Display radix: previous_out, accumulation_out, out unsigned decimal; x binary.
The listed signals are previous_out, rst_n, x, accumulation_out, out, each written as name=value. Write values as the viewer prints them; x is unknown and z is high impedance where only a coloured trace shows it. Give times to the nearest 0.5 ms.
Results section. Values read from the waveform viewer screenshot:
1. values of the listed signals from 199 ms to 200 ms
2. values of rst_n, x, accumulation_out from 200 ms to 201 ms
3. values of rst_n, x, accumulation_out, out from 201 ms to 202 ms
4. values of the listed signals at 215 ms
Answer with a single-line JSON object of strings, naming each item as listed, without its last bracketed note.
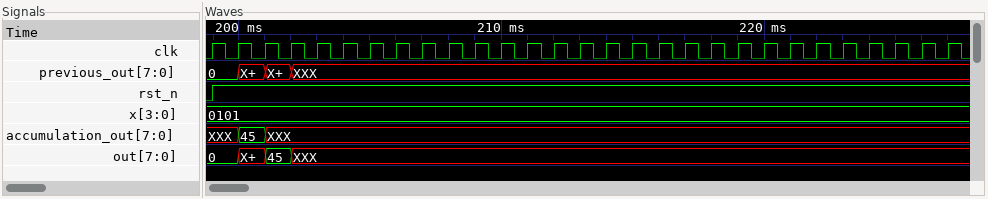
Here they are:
{"values of the listed signals from 199 ms to 200 ms": "previous_out=0, rst_n=1, x=0101, accumulation_out=XXX, out=0", "values of rst_n, x, accumulation_out from 200 ms to 201 ms": "rst_n=1, x=0101, accumulation_out=45", "values of rst_n, x, accumulation_out, out from 201 ms to 202 ms": "rst_n=1, x=0101, accumulation_out=XXX, out=45", "values of the listed signals at 215 ms": "previous_out=XXX, rst_n=1, x=0101, accumulation_out=XXX, out=XXX"}
